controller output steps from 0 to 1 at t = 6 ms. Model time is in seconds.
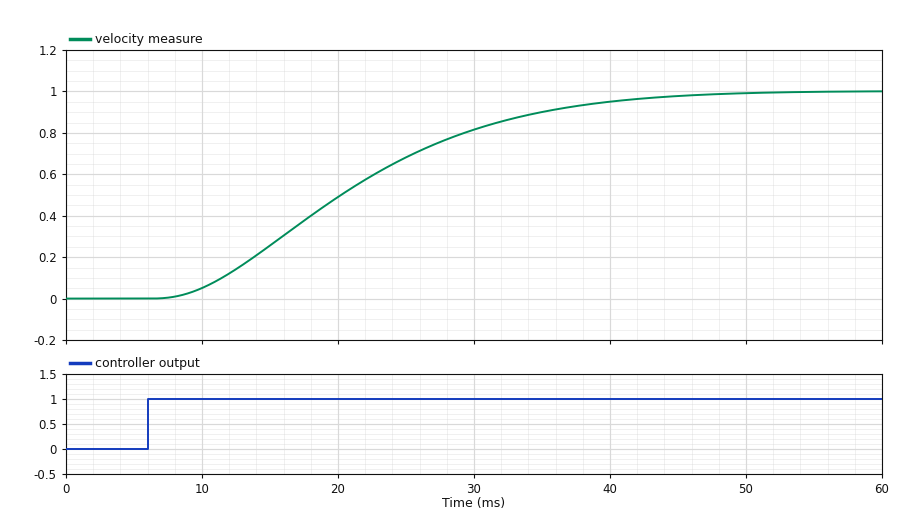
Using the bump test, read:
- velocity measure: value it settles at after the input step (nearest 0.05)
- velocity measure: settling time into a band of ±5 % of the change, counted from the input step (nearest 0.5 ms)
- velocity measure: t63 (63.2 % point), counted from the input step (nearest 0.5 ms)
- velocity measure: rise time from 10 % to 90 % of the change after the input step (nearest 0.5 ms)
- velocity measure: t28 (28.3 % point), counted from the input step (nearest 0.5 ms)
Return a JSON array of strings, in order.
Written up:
["1.00", "34.0 ms", "17.5 ms", "23.5 ms", "9.5 ms"]
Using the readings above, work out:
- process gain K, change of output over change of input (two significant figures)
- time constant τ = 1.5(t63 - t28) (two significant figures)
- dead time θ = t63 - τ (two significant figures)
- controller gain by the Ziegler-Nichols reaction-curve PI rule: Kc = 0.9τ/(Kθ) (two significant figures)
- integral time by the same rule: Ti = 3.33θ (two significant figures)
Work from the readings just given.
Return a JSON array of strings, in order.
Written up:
["1.0", "12 ms", "5.5 ms", "2.0", "18 ms"]
